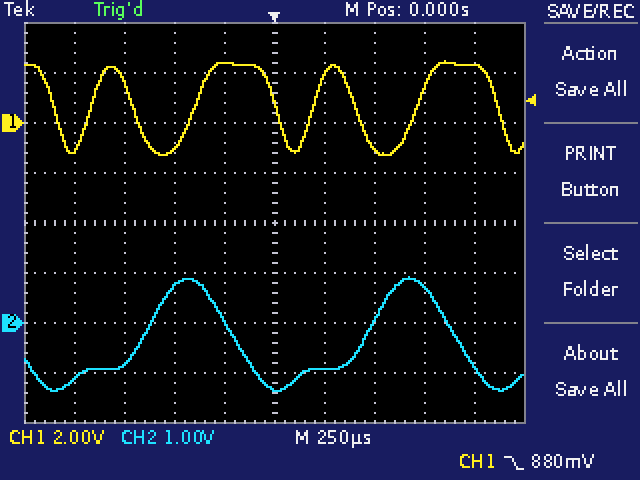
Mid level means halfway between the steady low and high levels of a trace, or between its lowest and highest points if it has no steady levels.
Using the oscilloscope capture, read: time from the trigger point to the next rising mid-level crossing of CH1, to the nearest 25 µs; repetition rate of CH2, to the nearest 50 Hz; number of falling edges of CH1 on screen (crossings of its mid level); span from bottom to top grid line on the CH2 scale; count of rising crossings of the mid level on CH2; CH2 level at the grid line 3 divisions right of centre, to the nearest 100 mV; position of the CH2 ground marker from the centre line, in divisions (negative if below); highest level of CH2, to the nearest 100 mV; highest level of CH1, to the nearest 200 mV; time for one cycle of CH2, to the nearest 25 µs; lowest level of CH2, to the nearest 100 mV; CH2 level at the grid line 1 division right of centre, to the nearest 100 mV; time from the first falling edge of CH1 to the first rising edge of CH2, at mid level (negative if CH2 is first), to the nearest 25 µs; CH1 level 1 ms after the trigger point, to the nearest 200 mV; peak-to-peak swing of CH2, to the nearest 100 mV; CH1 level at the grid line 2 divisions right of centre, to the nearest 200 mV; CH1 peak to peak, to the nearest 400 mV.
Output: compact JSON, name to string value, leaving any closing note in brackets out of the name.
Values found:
{"time from the trigger point to the next rising mid-level crossing of CH1, to the nearest 25 µs": "200 µs", "repetition rate of CH2, to the nearest 50 Hz": "900 Hz", "number of falling edges of CH1 on screen": "5", "span from bottom to top grid line on the CH2 scale": "8 V", "count of rising crossings of the mid level on CH2": "2", "CH2 level at the grid line 3 divisions right of centre, to the nearest 100 mV": "700 mV", "position of the CH2 ground marker from the centre line, in divisions": "-2.0 div", "highest level of CH2, to the nearest 100 mV": "900 mV", "highest level of CH1, to the nearest 200 mV": "2.4 V", "time for one cycle of CH2, to the nearest 25 µs": "1.100 ms", "lowest level of CH2, to the nearest 100 mV": "-1.4 V", "CH2 level at the grid line 1 division right of centre, to the nearest 100 mV": "-900 mV", "time from the first falling edge of CH1 to the first rising edge of CH2, at mid level (negative if CH2 is first), to the nearest 25 µs": "+450 µs", "CH1 level 1 ms after the trigger point, to the nearest 200 mV": "2.4 V", "peak-to-peak swing of CH2, to the nearest 100 mV": "2.3 V", "CH1 level at the grid line 2 divisions right of centre, to the nearest 200 mV": "-1.0 V", "CH1 peak to peak, to the nearest 400 mV": "3.6 V"}
